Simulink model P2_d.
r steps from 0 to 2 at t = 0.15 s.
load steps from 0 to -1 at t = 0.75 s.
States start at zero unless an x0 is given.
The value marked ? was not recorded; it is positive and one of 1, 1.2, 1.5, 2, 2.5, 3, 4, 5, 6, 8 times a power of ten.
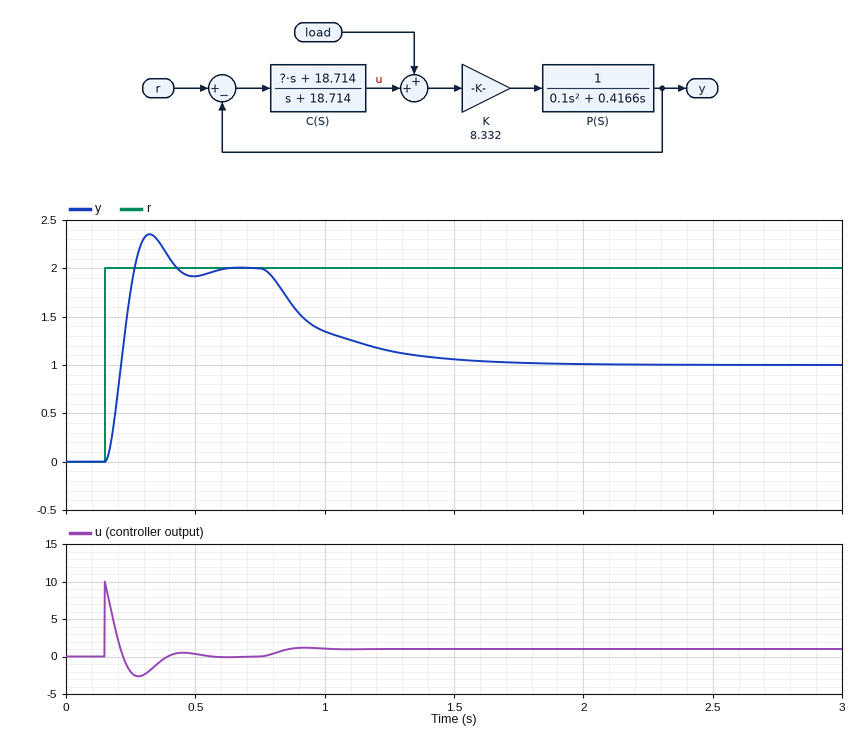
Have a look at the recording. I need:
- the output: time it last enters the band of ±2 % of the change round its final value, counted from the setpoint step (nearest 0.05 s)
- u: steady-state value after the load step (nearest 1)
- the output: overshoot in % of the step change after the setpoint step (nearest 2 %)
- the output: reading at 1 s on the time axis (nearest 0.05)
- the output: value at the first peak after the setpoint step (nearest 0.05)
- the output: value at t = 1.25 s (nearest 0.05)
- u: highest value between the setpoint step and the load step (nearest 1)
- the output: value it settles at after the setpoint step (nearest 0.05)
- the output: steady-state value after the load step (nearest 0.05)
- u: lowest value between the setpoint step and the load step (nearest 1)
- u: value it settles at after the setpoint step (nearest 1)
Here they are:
0.40 s
1
18 %
1.35
2.35
1.15
10
2.00
1.00
-3
0
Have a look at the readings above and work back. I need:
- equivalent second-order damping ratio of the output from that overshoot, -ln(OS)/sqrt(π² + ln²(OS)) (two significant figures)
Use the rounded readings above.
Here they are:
0.48
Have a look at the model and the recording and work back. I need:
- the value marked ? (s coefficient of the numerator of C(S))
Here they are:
5
